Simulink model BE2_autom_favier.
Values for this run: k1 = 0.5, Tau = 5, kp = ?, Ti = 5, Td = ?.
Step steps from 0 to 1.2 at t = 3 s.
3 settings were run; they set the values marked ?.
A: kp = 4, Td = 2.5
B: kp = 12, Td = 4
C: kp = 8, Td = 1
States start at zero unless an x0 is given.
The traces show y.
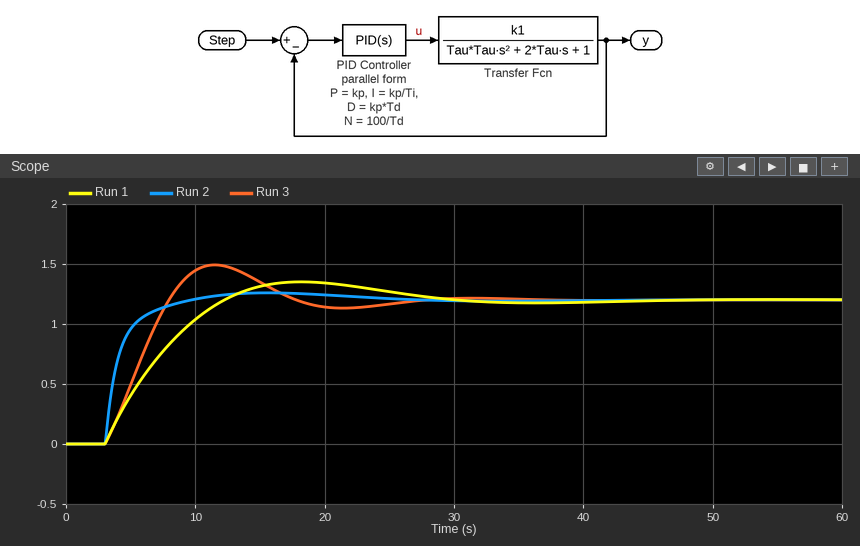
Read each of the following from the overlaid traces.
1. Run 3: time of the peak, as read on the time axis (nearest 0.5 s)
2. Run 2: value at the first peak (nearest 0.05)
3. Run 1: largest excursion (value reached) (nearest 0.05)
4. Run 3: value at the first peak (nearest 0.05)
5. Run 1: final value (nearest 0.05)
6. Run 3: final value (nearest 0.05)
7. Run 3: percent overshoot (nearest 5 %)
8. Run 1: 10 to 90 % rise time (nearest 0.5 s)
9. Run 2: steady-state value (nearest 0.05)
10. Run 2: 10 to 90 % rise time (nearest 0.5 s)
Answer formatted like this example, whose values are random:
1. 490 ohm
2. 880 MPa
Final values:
1. 11.5 s
2. 1.25
3. 1.35
4. 1.50
5. 1.20
6. 1.20
7. 25 %
8. 7.0 s
9. 1.20
10. 3.0 s
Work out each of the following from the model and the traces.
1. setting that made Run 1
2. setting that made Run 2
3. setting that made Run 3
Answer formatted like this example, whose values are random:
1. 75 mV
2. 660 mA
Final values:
1. A
2. B
3. C
